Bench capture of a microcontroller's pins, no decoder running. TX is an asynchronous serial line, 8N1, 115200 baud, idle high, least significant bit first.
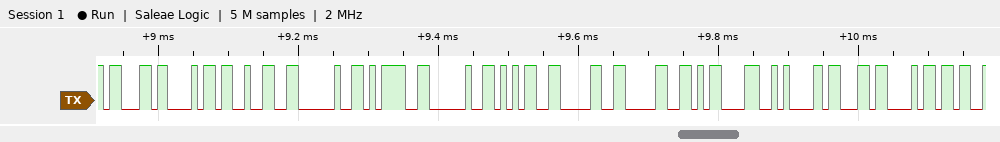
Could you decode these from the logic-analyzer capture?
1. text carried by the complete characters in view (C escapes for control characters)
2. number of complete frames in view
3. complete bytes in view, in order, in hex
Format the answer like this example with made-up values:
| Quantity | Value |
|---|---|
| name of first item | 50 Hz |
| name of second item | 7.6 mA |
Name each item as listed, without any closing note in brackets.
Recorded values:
| Quantity | Value |
|---|---|
| text carried by the complete characters in view | "ch2 = 500\r\nch" |
| number of complete frames in view | 13 |
| complete bytes in view, in order, in hex | 63 68 32 20 3D 20 35 30 30 0D 0A 63 68 |
